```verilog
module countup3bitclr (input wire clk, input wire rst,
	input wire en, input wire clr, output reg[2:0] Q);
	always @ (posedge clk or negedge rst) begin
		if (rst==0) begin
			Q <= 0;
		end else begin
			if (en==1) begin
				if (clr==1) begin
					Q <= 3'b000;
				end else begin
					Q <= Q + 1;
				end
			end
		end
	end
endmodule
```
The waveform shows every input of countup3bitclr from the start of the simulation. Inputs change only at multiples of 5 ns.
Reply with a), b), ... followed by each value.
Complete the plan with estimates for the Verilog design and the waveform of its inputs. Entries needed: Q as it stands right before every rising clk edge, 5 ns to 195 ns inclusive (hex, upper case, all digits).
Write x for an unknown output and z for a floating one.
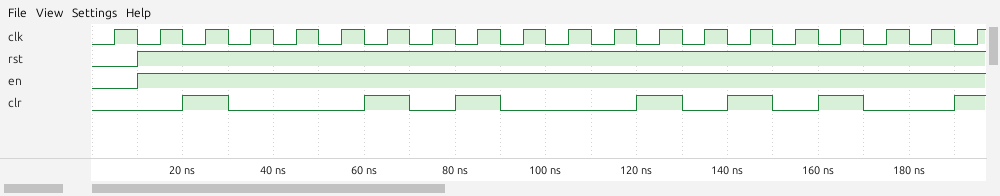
a) 0, 0, 1, 0, 1, 2, 3, 0, 1, 0, 1, 2, 3, 0, 1, 0, 1, 0, 1, 2
